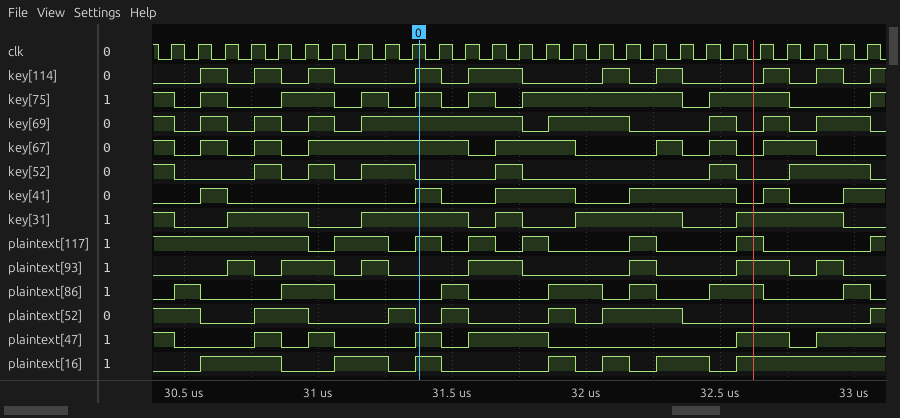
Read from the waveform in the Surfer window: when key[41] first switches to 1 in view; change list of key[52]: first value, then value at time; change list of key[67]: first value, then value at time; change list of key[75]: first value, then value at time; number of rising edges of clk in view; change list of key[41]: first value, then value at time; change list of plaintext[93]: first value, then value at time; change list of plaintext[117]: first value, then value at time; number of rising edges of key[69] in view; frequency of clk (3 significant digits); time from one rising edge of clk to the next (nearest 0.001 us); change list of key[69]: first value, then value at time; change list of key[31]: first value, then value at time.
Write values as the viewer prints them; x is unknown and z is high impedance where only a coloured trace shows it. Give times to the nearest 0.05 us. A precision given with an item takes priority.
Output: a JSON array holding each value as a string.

["30.55 us", "1, 0 at 30.45 us, 1 at 30.75 us, 0 at 30.85 us, 1 at 30.95 us, 0 at 31.05 us, 1 at 31.15 us, 0 at 31.35 us, 1 at 31.65 us, 0 at 31.75 us, 1 at 32.45 us, 0 at 32.55 us, 1 at 32.75 us, 0 at 33.05 us", "1, 0 at 30.45 us, 1 at 30.55 us, 0 at 30.65 us, 1 at 30.75 us, 0 at 30.85 us, 1 at 30.95 us, 0 at 31.55 us, 1 at 31.65 us, 0 at 31.95 us, 1 at 32.25 us, 0 at 32.35 us, 1 at 32.45 us, 0 at 32.55 us, 1 at 32.65 us, 0 at 32.85 us", "1, 0 at 30.45 us, 1 at 30.55 us, 0 at 30.65 us, 1 at 30.85 us, 0 at 31.05 us, 1 at 31.15 us, 0 at 31.25 us, 1 at 31.35 us, 0 at 31.45 us, 1 at 31.55 us, 0 at 31.65 us, 1 at 31.75 us, 0 at 32.35 us, 1 at 32.45 us, 0 at 32.75 us, 1 at 33.05 us", "27", "0, 1 at 30.55 us, 0 at 30.65 us, 1 at 31.35 us, 0 at 31.45 us, 1 at 31.65 us, 0 at 31.95 us, 1 at 32.15 us, 0 at 32.55 us, 1 at 32.65 us, 0 at 32.75 us, 1 at 32.95 us", "0, 1 at 30.65 us, 0 at 30.75 us, 1 at 30.85 us, 0 at 31.05 us, 1 at 31.15 us, 0 at 31.25 us, 1 at 31.55 us, 0 at 31.75 us, 1 at 32.15 us, 0 at 32.25 us, 1 at 32.55 us, 0 at 32.75 us, 1 at 32.85 us, 0 at 32.95 us", "1, 0 at 30.95 us, 1 at 31.05 us, 0 at 31.25 us, 1 at 31.35 us, 0 at 31.45 us, 1 at 31.55 us, 0 at 31.65 us, 1 at 31.75 us, 0 at 31.85 us, 1 at 32.15 us, 0 at 32.25 us, 1 at 32.55 us, 0 at 32.65 us, 1 at 33.05 us", "8", "10.0 MHz", "0.1 us", "1, 0 at 30.45 us, 1 at 30.55 us, 0 at 30.65 us, 1 at 30.75 us, 0 at 30.85 us, 1 at 30.95 us, 0 at 31.05 us, 1 at 31.15 us, 0 at 31.75 us, 1 at 31.85 us, 0 at 32.15 us, 1 at 32.45 us, 0 at 32.55 us, 1 at 32.65 us, 0 at 32.75 us, 1 at 32.85 us, 0 at 33.05 us", "1, 0 at 30.45 us, 1 at 30.65 us, 0 at 30.95 us, 1 at 31.15 us, 0 at 31.55 us, 1 at 31.65 us, 0 at 31.75 us, 1 at 31.95 us, 0 at 32.35 us, 1 at 32.55 us, 0 at 32.95 us"]
